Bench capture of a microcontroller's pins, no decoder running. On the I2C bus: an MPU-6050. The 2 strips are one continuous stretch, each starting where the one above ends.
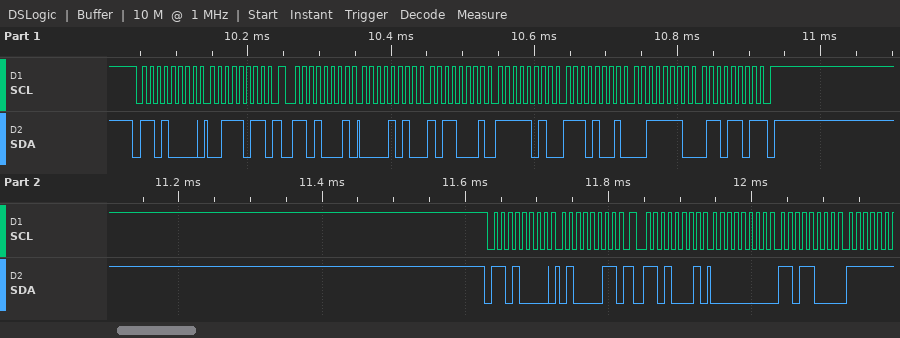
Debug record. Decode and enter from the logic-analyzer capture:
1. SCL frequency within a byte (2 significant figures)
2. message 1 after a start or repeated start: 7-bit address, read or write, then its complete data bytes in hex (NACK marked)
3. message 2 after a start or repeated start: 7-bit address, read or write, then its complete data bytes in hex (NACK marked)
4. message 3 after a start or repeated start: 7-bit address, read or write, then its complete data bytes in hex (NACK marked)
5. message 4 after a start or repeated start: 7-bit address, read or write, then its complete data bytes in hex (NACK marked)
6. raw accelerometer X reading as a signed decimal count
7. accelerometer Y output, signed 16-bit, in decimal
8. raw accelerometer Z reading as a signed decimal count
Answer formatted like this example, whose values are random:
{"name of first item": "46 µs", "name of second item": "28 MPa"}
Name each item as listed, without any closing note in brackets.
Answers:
{"SCL frequency within a byte": "100 kHz", "message 1 after a start or repeated start: 7-bit address, read or write, then its complete data bytes in hex": "0x68 write: 3B", "message 2 after a start or repeated start: 7-bit address, read or write, then its complete data bytes in hex": "0x68 read: 0A B1 FA E9 3E 6D NACK", "message 3 after a start or repeated start: 7-bit address, read or write, then its complete data bytes in hex": "0x68 write: 43", "message 4 after a start or repeated start: 7-bit address, read or write, then its complete data bytes in hex": "0x68 read: 00 D8", "raw accelerometer X reading as a signed decimal count": "2737", "accelerometer Y output, signed 16-bit, in decimal": "-1303", "raw accelerometer Z reading as a signed decimal count": "15981"}
